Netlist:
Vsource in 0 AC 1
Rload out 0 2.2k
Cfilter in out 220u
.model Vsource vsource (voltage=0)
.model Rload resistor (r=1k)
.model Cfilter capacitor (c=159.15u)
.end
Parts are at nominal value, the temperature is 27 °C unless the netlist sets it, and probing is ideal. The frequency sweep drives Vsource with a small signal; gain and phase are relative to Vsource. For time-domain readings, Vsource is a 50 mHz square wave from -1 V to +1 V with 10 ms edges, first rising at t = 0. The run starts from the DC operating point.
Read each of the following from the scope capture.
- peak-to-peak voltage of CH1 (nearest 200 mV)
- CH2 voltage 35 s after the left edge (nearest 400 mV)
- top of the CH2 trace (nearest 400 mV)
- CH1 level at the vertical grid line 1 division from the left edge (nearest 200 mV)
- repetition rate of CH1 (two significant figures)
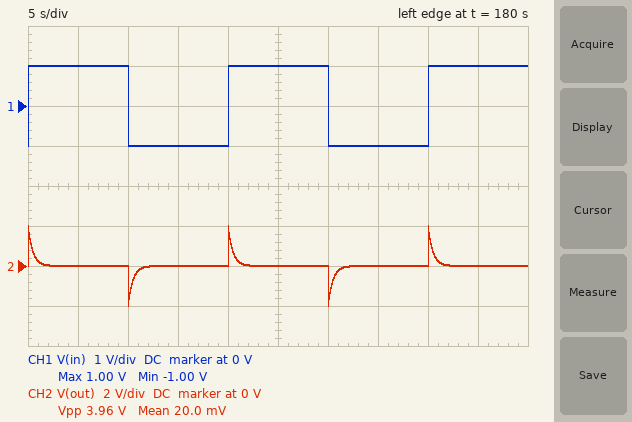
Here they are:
2.0 V
0 V
2.0 V
1.0 V
50 mHz
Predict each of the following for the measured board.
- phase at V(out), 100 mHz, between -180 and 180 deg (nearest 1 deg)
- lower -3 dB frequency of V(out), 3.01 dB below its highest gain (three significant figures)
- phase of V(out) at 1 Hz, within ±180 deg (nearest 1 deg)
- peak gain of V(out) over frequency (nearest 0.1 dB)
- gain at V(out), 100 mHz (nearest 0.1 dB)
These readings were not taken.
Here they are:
73 deg
329 mHz
18 deg
0 dB
-10.7 dB
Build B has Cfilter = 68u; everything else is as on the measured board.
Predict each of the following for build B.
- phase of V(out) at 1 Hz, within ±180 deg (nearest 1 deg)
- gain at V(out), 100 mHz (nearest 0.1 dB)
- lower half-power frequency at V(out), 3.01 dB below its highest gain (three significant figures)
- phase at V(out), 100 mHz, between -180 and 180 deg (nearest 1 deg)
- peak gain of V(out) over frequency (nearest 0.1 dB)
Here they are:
47 deg
-20.6 dB
1.06 Hz
85 deg
0 dB
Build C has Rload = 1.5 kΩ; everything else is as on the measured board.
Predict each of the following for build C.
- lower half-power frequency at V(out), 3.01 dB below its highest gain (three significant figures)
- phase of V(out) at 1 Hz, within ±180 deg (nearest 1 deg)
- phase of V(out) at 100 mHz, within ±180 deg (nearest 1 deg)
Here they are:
482 mHz
26 deg
78 deg
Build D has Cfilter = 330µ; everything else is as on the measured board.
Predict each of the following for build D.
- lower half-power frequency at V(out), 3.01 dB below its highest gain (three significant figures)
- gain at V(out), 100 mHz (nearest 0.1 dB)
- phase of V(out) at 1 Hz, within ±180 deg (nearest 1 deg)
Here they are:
219 mHz
-7.6 dB
12 deg
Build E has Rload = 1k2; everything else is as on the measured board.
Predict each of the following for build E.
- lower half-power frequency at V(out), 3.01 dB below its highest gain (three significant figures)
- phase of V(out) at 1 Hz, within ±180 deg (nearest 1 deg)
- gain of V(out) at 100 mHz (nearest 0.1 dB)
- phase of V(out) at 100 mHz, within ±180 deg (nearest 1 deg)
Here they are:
603 mHz
31 deg
-15.7 dB
81 deg
